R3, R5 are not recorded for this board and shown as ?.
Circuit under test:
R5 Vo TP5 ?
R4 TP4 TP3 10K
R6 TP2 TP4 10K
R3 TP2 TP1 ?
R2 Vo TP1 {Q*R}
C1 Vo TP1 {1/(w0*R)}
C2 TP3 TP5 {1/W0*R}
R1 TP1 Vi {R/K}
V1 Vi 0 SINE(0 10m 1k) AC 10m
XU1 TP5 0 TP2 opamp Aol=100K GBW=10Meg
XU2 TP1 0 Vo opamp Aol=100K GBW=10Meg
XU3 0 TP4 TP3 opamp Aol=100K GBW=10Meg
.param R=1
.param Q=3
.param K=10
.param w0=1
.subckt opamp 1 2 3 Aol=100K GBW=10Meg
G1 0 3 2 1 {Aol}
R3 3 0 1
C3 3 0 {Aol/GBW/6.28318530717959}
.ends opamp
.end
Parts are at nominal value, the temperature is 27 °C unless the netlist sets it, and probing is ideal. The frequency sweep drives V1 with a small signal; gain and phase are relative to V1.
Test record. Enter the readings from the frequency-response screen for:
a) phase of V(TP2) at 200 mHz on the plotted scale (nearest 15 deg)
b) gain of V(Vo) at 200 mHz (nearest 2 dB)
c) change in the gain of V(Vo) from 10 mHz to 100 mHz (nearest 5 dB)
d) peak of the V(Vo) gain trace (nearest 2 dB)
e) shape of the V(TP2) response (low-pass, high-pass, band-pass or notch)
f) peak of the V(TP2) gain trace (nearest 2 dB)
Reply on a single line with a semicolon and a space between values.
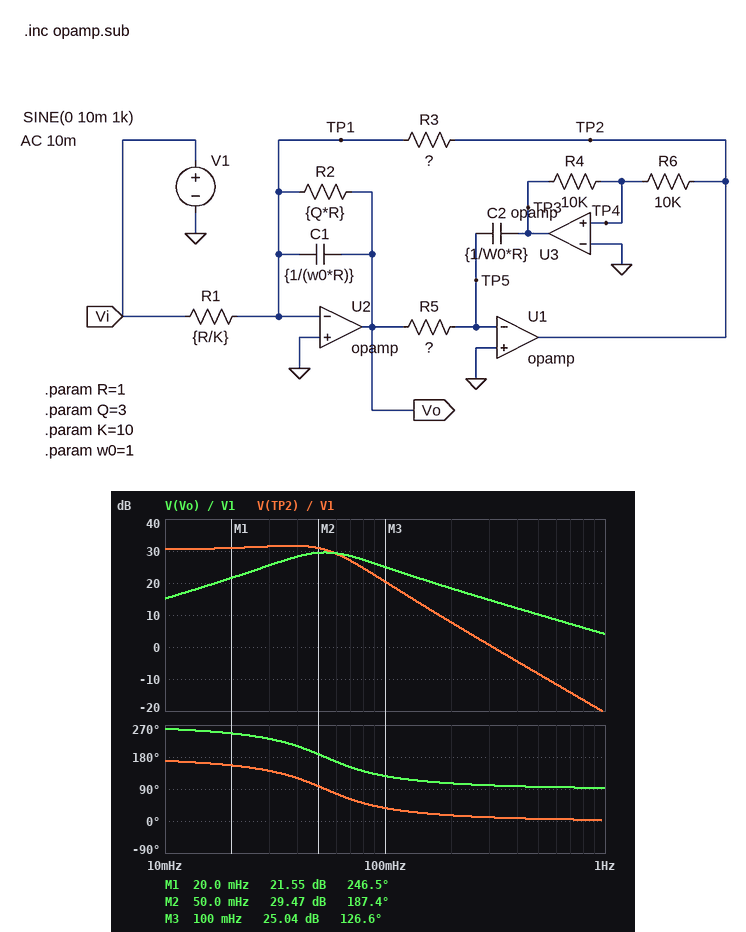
15 deg; 18 dB; 10 dB; 30 dB; low-pass; 32 dB
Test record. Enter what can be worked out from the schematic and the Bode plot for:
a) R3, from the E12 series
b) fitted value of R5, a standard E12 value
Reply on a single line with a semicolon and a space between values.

3.3 Ω; 2.7 Ω
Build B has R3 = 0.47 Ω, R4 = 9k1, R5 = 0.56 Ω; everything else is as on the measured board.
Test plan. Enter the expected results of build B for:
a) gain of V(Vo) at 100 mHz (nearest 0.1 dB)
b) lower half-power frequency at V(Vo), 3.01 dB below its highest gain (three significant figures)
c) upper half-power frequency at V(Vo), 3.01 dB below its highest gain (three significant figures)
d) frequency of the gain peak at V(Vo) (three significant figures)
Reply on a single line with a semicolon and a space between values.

4.4 dB; 300 mHz; 353 mHz; 325 mHz
